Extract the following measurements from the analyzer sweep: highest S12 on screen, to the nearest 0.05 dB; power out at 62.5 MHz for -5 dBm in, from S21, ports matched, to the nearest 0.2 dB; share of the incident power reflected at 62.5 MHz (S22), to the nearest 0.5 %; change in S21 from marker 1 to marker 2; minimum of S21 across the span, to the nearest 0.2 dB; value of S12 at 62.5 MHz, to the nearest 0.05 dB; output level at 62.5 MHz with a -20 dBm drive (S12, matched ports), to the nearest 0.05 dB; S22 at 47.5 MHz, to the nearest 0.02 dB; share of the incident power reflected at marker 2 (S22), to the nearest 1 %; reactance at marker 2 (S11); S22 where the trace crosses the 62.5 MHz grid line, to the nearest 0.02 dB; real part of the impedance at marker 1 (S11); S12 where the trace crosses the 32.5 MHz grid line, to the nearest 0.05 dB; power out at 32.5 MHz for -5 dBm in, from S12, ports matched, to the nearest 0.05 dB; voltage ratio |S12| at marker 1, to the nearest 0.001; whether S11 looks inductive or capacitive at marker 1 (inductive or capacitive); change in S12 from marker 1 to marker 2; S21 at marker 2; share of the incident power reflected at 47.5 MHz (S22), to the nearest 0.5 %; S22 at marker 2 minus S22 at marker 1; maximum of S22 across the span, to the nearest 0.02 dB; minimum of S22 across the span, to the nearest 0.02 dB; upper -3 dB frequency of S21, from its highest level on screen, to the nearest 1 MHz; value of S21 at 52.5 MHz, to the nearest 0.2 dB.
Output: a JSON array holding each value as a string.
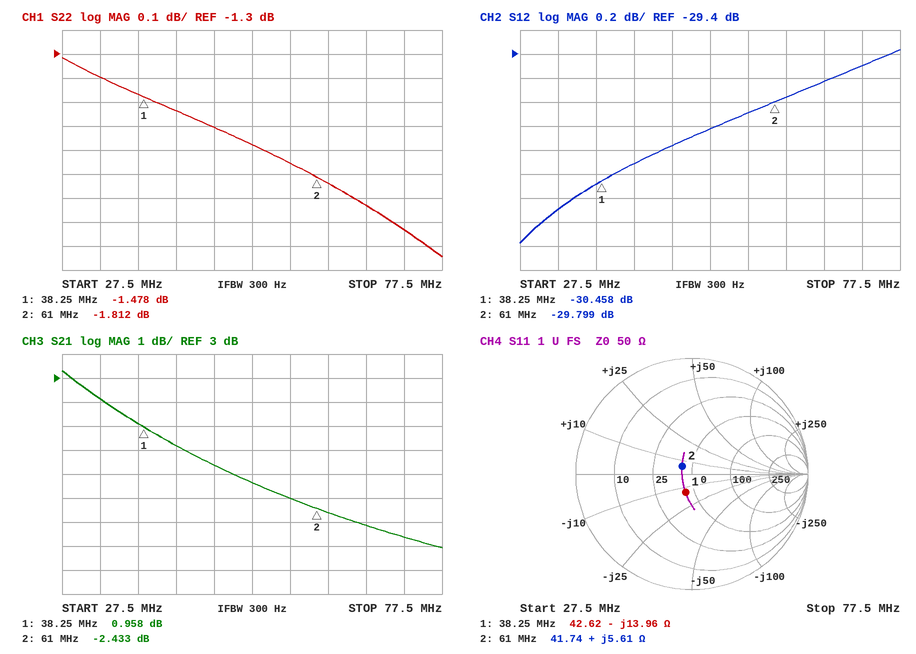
["-29.35 dB", "-7.6 dBm", "65.5 %", "-3.391 dB", "-4.0 dB", "-29.75 dB", "-49.75 dBm", "-1.60 dB", "66 %", "+5.61 Ω", "-1.84 dB", "42.62 Ω", "-30.70 dB", "-35.70 dBm", "0.030", "capacitive", "0.659 dB", "-2.433 dB", "69.0 %", "-0.334 dB", "-1.32 dB", "-2.14 dB", "42 MHz", "-1.4 dB"]
